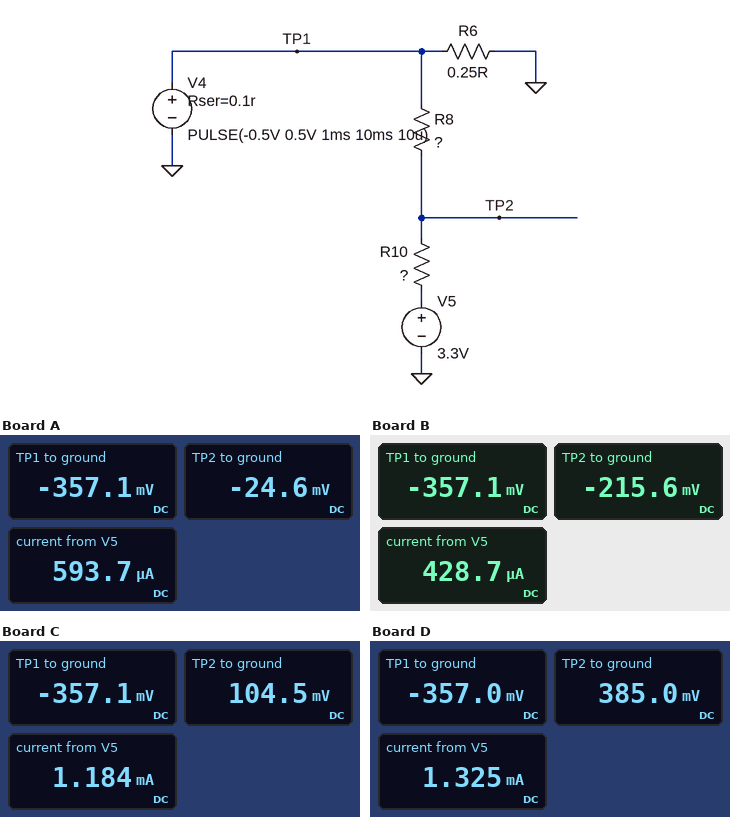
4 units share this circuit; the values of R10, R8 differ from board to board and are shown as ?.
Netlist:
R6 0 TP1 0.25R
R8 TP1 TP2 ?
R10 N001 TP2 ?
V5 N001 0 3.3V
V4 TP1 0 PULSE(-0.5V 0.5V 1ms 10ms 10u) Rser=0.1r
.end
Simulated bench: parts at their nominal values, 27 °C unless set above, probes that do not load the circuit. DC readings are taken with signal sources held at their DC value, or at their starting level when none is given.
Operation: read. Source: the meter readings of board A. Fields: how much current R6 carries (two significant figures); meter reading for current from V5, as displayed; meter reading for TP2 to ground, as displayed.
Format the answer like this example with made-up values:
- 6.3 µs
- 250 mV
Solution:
- 1.4 A
- 593.7 µA
- -24.6 mV
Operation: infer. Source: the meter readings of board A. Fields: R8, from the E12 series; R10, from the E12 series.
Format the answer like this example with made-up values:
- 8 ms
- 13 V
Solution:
- 560 Ω
- 5.6 kΩ
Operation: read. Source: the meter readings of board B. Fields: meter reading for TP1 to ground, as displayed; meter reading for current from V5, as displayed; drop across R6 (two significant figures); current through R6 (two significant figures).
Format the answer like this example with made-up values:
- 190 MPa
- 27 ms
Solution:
- -357.1 mV
- 428.7 µA
- 360 mV
- 1.4 A
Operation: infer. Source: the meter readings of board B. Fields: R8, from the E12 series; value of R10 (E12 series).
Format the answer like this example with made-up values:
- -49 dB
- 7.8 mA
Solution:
- 330 Ω
- 8.2 kΩ
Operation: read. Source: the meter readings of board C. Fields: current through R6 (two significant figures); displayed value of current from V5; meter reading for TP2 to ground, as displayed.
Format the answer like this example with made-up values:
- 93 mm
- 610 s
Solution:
- 1.4 A
- 1.184 mA
- 104.5 mV
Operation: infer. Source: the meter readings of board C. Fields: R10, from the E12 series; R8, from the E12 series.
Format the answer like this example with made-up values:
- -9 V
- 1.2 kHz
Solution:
- 2.7 kΩ
- 390 Ω
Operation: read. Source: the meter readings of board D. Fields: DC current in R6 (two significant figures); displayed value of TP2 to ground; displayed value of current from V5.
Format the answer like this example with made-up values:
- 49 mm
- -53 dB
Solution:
- 1.4 A
- 385.0 mV
- 1.325 mA
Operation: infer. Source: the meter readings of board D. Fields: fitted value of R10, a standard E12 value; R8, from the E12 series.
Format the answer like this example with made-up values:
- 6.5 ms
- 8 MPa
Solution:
- 2.2 kΩ
- 560 Ω
